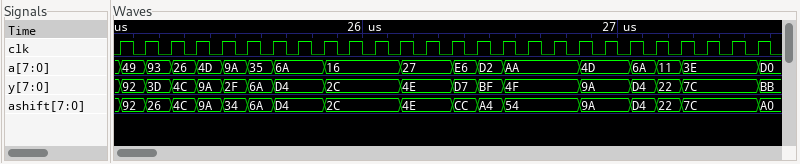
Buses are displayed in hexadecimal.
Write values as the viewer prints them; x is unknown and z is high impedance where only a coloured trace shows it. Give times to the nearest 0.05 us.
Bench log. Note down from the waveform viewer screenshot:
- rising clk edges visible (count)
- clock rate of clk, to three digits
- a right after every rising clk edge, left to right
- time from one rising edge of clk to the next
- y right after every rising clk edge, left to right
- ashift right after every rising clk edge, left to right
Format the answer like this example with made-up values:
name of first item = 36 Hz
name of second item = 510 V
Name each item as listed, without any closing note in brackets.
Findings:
rising clk edges visible = 26
clock rate of clk, to three digits = 10.0 MHz
a right after every rising clk edge, left to right = 49, 93, 26, 4D, 9A, 35, 6A, 6A, 16, 16, 16, 27, 27, E6, D2, AA, AA, AA, 4D, 4D, 6A, 11, 3E, 3E, 3E, D0
time from one rising edge of clk to the next = 0.1 us
y right after every rising clk edge, left to right = 92, 3D, 4C, 9A, 2F, 6A, D4, D4, 2C, 2C, 2C, 4E, 4E, D7, BF, 4F, 4F, 4F, 9A, 9A, D4, 22, 7C, 7C, 7C, BB
ashift right after every rising clk edge, left to right = 92, 26, 4C, 9A, 34, 6A, D4, D4, 2C, 2C, 2C, 4E, 4E, CC, A4, 54, 54, 54, 9A, 9A, D4, 22, 7C, 7C, 7C, A0
